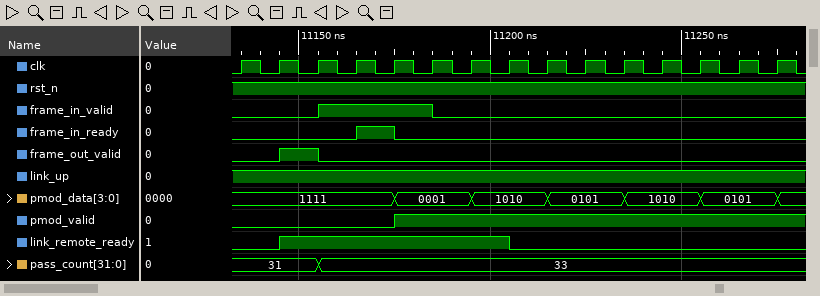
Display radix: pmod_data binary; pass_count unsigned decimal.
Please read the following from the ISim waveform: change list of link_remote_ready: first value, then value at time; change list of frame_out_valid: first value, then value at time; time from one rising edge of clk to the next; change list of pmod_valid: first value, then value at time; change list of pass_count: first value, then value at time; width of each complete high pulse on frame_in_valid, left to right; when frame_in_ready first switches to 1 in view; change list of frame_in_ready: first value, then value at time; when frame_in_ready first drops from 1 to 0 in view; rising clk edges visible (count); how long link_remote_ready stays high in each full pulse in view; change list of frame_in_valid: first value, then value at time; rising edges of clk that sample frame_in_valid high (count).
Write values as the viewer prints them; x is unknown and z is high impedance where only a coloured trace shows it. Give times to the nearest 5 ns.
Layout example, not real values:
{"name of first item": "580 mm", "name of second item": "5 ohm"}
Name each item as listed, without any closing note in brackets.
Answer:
{"change list of link_remote_ready: first value, then value at time": "0, 1 at 11145 ns, 0 at 11205 ns", "change list of frame_out_valid: first value, then value at time": "0, 1 at 11145 ns, 0 at 11155 ns", "time from one rising edge of clk to the next": "10 ns", "change list of pmod_valid: first value, then value at time": "0, 1 at 11175 ns", "change list of pass_count: first value, then value at time": "31, 33 at 11155 ns", "width of each complete high pulse on frame_in_valid, left to right": "30 ns", "when frame_in_ready first switches to 1 in view": "11165 ns", "change list of frame_in_ready: first value, then value at time": "0, 1 at 11165 ns, 0 at 11175 ns", "when frame_in_ready first drops from 1 to 0 in view": "11175 ns", "rising clk edges visible": "15", "how long link_remote_ready stays high in each full pulse in view": "60 ns", "change list of frame_in_valid: first value, then value at time": "0, 1 at 11155 ns, 0 at 11185 ns", "rising edges of clk that sample frame_in_valid high": "3"}
